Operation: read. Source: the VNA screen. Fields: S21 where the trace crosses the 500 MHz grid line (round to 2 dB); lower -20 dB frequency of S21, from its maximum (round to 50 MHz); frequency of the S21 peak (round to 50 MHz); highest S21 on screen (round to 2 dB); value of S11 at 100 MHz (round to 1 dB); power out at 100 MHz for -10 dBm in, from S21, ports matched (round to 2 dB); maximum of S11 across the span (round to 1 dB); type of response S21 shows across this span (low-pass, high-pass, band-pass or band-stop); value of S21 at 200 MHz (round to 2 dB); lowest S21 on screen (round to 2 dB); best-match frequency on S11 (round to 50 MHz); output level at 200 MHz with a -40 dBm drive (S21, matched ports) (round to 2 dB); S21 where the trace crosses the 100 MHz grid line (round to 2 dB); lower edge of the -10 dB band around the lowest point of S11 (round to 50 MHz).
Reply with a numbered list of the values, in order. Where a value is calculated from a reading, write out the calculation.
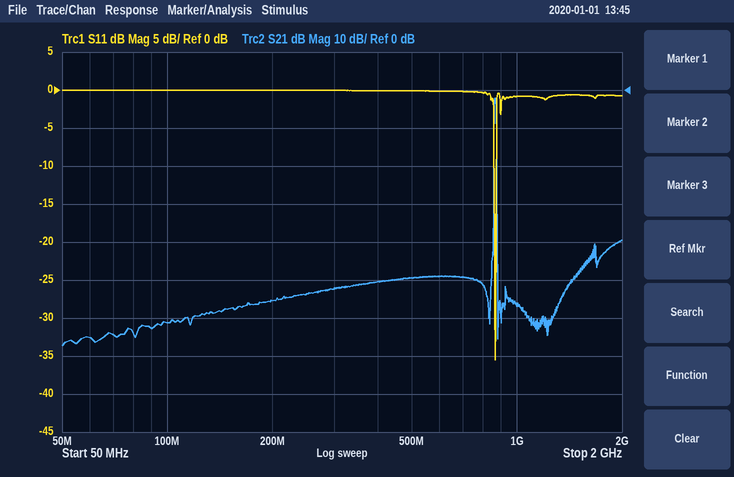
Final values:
1. -50 dB
2. 850 MHz
3. 850 MHz
4. -2 dB
5. 0 dB
6. -10 dBm + (-62 dB) = -72 dBm
7. 0 dB
8. band-pass
9. -56 dB
10. -68 dB
11. 850 MHz
12. -40 dBm + (-56 dB) = -96 dBm
13. -62 dB
14. 850 MHz
